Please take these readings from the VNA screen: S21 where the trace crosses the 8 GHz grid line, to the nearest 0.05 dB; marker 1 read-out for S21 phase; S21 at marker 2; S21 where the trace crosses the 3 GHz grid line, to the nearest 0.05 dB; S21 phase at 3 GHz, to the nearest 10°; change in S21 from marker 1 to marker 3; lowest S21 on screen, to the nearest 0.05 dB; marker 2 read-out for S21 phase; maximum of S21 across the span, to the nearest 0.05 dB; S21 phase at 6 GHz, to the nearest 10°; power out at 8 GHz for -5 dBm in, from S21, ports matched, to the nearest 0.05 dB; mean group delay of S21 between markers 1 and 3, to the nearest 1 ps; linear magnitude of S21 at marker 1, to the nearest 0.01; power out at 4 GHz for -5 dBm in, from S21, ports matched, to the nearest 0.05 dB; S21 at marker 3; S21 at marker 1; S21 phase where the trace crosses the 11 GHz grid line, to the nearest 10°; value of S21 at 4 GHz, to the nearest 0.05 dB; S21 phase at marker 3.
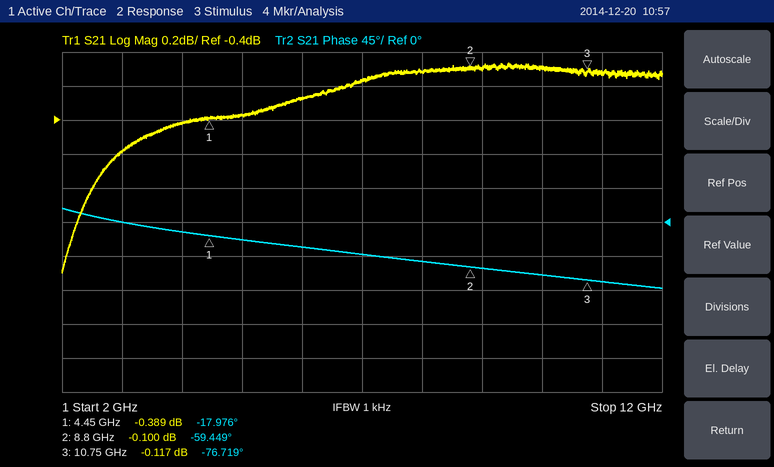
-0.10 dB
-17.976°
-0.100 dB
-0.60 dB
0°
0.272 dB
-1.30 dB
-59.449°
-0.05 dB
-30°
-5.10 dBm
26 ps
0.96
-5.40 dBm
-0.117 dB
-0.389 dB
-80°
-0.40 dB
-76.719°
